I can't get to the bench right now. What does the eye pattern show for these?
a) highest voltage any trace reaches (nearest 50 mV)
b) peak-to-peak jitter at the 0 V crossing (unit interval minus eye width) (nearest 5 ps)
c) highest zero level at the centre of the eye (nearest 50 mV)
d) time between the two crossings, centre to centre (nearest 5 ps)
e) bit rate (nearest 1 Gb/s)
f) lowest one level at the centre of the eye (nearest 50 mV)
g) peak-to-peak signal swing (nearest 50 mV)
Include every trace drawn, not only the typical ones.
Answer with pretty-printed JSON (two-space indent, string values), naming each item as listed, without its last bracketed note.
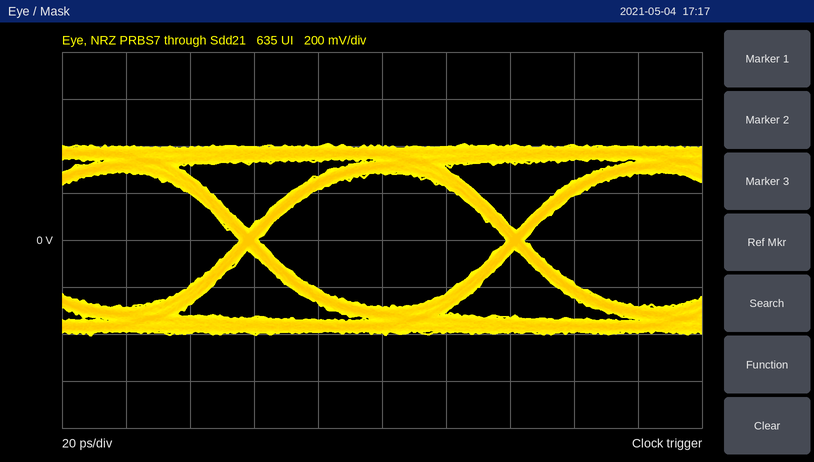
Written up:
{
  "highest voltage any trace reaches": "400 mV",
  "peak-to-peak jitter at the 0 V crossing (unit interval minus eye width)": "5 ps",
  "highest zero level at the centre of the eye": "-300 mV",
  "time between the two crossings, centre to centre": "85 ps",
  "bit rate": "12 Gb/s",
  "lowest one level at the centre of the eye": "300 mV",
  "peak-to-peak signal swing": "800 mV"
}
